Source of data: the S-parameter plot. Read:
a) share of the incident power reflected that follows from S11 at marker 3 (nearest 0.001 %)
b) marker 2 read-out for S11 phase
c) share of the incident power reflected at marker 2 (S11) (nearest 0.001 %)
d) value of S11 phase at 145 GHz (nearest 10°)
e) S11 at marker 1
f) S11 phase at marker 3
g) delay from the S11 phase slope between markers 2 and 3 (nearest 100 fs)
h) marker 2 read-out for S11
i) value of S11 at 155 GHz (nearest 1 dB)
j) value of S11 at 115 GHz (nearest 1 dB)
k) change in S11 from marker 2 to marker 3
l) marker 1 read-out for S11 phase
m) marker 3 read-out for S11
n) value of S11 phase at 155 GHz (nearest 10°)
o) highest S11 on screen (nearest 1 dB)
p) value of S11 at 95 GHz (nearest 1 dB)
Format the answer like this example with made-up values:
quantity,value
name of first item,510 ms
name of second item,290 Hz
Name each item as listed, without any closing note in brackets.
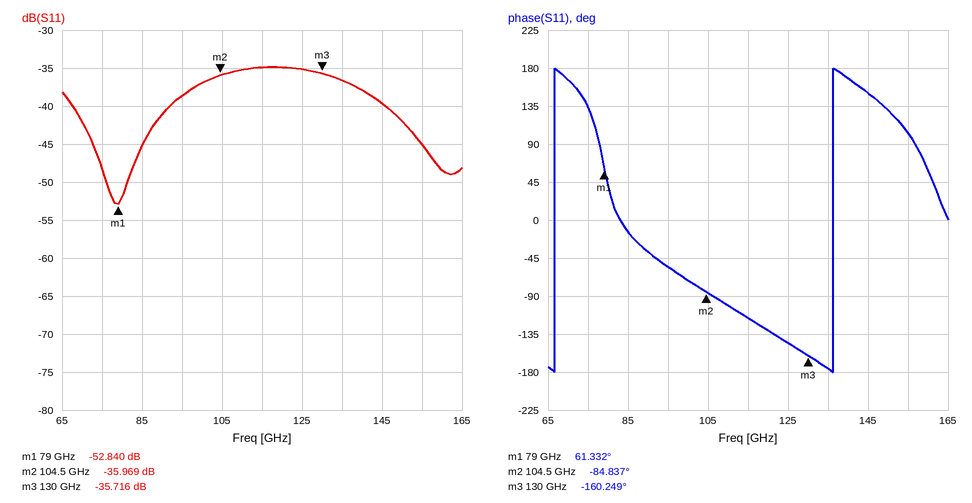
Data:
quantity,value
share of the incident power reflected that follows from S11 at marker 3,0.027 %
marker 2 read-out for S11 phase,-84.837°
share of the incident power reflected at marker 2 (S11),0.025 %
value of S11 phase at 145 GHz,150°
S11 at marker 1,-52.840 dB
S11 phase at marker 3,-160.249°
delay from the S11 phase slope between markers 2 and 3,8.2 ps
marker 2 read-out for S11,-35.969 dB
value of S11 at 155 GHz,-45 dB
value of S11 at 115 GHz,-35 dB
change in S11 from marker 2 to marker 3,0.253 dB
marker 1 read-out for S11 phase,61.332°
marker 3 read-out for S11,-35.716 dB
value of S11 phase at 155 GHz,100°
highest S11 on screen,-35 dB
value of S11 at 95 GHz,-39 dB
